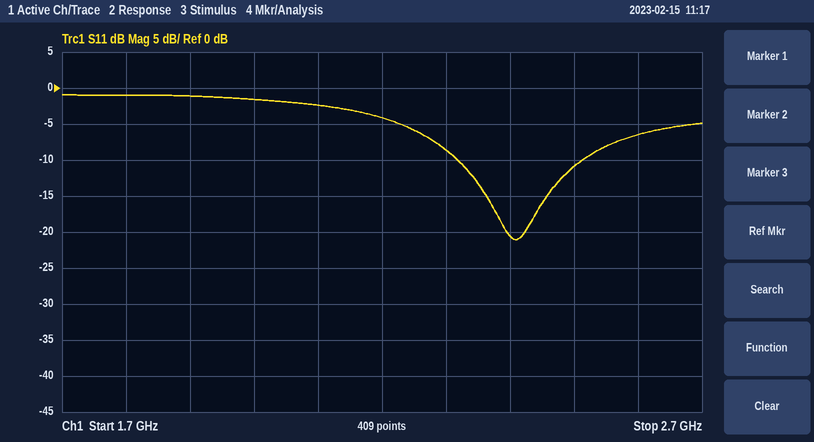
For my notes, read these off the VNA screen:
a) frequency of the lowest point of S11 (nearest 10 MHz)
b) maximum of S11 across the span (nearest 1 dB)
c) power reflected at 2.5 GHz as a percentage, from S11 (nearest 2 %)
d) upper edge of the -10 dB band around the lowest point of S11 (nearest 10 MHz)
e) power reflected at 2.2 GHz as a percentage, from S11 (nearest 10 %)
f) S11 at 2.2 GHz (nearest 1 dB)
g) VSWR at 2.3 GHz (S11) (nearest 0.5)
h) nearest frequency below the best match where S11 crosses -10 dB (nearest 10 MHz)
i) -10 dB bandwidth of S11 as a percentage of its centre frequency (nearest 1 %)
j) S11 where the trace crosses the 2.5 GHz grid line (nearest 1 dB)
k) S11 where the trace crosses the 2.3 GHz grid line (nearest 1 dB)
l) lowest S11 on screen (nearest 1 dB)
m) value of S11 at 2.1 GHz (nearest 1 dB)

2.41 GHz
-1 dB
8 %
2.51 GHz
40 %
-4 dB
2.0
2.32 GHz
8 %
-11 dB
-9 dB
-21 dB
-2 dB
